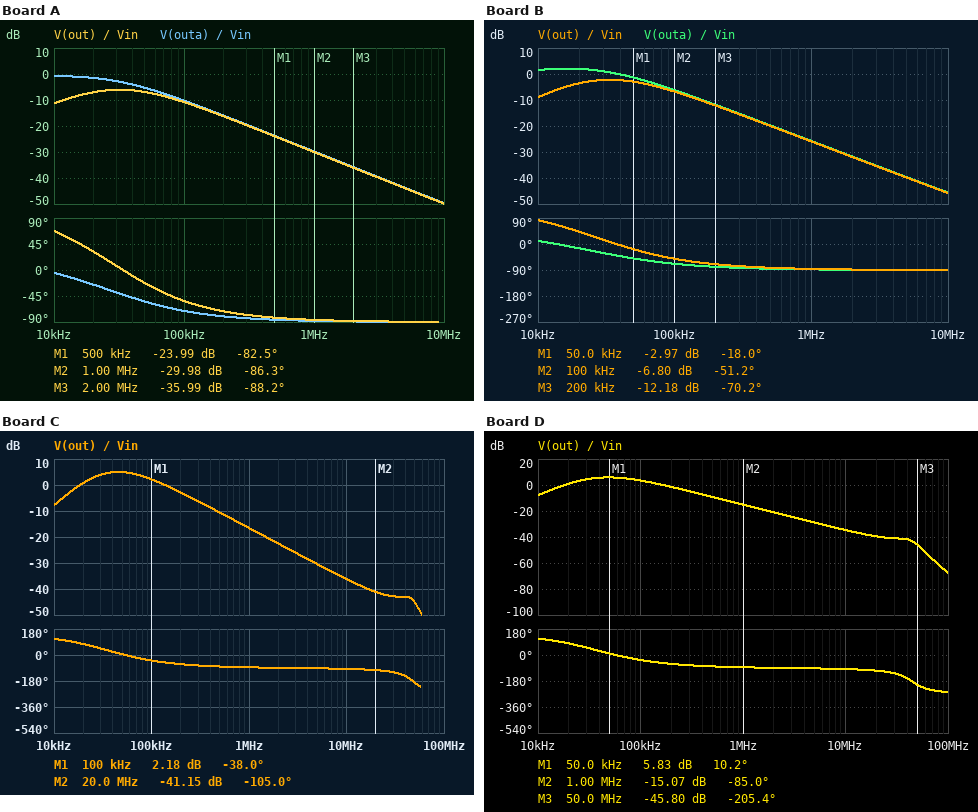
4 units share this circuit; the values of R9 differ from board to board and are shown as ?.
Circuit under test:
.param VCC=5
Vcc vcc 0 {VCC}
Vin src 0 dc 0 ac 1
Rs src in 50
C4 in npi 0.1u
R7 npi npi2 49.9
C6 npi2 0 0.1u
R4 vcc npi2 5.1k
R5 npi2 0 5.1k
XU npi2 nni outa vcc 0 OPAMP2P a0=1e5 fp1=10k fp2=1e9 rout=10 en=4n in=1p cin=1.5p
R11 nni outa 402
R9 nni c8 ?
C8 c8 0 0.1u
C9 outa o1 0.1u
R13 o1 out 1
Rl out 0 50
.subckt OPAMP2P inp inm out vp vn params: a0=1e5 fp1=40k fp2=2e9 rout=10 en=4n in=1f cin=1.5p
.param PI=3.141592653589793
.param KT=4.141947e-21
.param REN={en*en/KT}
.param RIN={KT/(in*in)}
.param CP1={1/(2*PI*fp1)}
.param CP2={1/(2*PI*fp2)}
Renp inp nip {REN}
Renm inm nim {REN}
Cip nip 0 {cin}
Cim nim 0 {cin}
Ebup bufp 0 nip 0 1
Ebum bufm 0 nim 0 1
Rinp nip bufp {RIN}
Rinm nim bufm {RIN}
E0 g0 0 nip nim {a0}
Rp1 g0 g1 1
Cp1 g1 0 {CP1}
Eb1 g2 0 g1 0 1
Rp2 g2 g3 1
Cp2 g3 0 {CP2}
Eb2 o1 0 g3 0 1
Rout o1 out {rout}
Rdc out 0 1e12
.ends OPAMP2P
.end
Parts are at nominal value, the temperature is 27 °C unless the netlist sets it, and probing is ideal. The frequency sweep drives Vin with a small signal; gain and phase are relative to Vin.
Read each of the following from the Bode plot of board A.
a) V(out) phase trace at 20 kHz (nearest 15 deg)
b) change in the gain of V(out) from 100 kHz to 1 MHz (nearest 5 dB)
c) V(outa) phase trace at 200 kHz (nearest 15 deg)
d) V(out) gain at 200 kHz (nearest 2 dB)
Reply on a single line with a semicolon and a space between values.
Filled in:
30 deg; -20 dB; -75 deg; -16 dB
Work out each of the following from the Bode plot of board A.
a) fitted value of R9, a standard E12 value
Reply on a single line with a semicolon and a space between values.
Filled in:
390 Ω
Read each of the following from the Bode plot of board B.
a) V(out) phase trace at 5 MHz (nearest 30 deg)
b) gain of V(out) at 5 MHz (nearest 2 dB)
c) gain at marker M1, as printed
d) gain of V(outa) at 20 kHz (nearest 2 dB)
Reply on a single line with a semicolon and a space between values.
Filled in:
-90 deg; -40 dB; -2.97 dB; 2 dB
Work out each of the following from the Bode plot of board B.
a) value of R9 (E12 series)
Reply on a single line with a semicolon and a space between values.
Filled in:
180 Ω
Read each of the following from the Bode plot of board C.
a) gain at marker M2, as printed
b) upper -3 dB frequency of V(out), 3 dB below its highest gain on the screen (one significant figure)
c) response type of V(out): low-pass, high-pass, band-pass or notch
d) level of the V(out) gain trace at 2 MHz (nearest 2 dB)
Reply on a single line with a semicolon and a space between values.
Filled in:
-41.15 dB; 100 kHz; band-pass; -22 dB
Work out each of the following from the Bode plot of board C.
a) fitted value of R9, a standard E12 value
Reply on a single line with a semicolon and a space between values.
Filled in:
47 Ω
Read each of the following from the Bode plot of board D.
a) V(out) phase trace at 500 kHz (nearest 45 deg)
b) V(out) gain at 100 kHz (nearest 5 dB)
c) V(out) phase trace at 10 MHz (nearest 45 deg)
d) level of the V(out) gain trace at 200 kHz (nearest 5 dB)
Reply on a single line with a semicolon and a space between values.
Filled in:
-90 deg; 5 dB; -90 deg; 0 dB
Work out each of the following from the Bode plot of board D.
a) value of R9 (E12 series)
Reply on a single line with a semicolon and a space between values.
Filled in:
39 Ω
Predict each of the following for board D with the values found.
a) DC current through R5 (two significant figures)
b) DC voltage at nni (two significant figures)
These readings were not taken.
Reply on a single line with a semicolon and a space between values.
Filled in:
490 µA; 2.5 V
